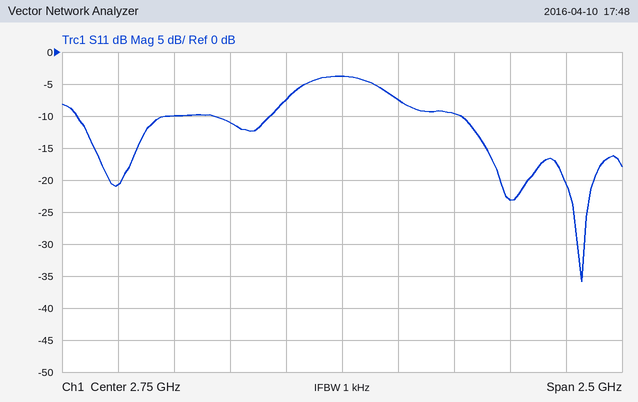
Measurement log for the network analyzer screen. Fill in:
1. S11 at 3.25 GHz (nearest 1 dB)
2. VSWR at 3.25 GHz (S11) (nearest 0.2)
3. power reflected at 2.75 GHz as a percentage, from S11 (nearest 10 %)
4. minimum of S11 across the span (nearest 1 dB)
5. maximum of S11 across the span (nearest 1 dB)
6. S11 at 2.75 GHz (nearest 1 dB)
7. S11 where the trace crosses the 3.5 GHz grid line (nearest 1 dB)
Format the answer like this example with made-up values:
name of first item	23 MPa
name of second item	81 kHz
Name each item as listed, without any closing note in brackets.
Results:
S11 at 3.25 GHz	-10 dB
VSWR at 3.25 GHz (S11)	2.0
power reflected at 2.75 GHz as a percentage, from S11	40 %
minimum of S11 across the span	-36 dB
maximum of S11 across the span	-4 dB
S11 at 2.75 GHz	-4 dB
S11 where the trace crosses the 3.5 GHz grid line	-23 dB
